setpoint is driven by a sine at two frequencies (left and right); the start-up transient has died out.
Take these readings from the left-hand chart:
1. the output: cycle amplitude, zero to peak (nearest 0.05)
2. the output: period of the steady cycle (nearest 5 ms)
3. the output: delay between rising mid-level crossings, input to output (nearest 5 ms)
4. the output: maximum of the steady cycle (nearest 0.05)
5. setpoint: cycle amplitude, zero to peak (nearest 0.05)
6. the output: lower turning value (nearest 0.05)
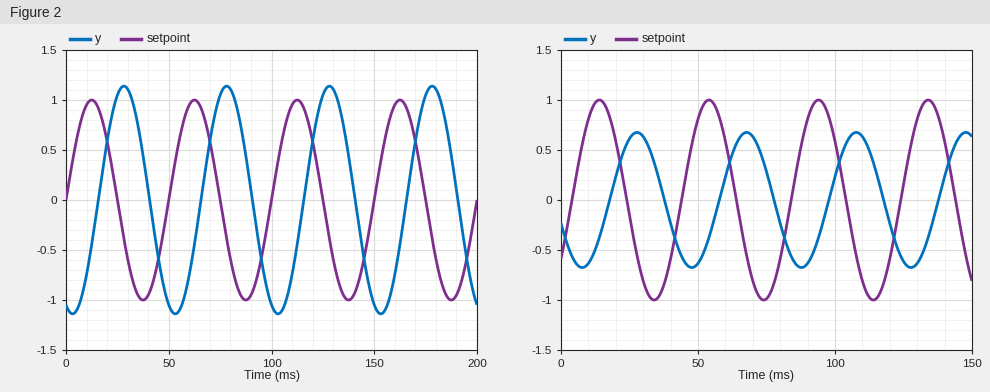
1.15
50 ms
15 ms
1.15
1.00
-1.15
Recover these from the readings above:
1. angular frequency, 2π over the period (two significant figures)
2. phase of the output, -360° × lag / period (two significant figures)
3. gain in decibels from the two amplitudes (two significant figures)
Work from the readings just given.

0.13 rad/ms
-110°
1.2 dB
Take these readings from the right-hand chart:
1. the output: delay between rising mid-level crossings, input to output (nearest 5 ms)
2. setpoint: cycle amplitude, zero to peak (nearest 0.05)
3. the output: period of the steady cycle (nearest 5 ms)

15 ms
1.00
40 ms
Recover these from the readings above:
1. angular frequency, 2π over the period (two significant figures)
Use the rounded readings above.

0.16 rad/ms
